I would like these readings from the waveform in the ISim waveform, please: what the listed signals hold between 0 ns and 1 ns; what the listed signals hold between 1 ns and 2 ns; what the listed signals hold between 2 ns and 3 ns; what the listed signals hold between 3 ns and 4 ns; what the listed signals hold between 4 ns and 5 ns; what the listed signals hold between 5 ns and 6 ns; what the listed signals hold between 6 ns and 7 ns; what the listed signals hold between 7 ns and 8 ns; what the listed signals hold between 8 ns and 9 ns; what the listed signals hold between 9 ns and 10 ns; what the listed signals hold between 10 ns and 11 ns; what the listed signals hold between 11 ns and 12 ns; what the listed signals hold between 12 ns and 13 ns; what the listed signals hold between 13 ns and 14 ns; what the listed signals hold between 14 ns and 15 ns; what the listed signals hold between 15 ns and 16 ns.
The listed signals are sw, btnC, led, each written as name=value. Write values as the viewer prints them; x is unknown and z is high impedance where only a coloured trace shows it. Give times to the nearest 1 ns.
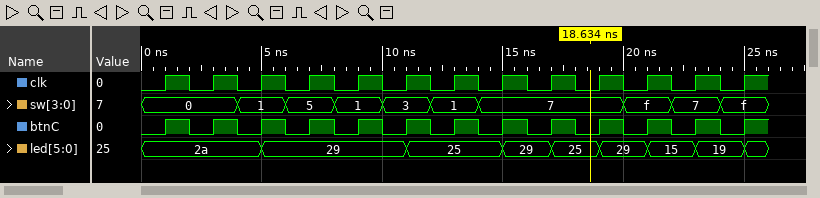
sw=0, btnC=0, led=2a
sw=0, btnC=1, led=2a
sw=0, btnC=0, led=2a
sw=0, btnC=1, led=2a
sw=1, btnC=0, led=2a
sw=1, btnC=1, led=29
sw=5, btnC=0, led=29
sw=5, btnC=1, led=29
sw=1, btnC=0, led=29
sw=1, btnC=1, led=29
sw=3, btnC=0, led=29
sw=3, btnC=1, led=25
sw=1, btnC=0, led=25
sw=1, btnC=1, led=25
sw=7, btnC=0, led=25
sw=7, btnC=1, led=29
